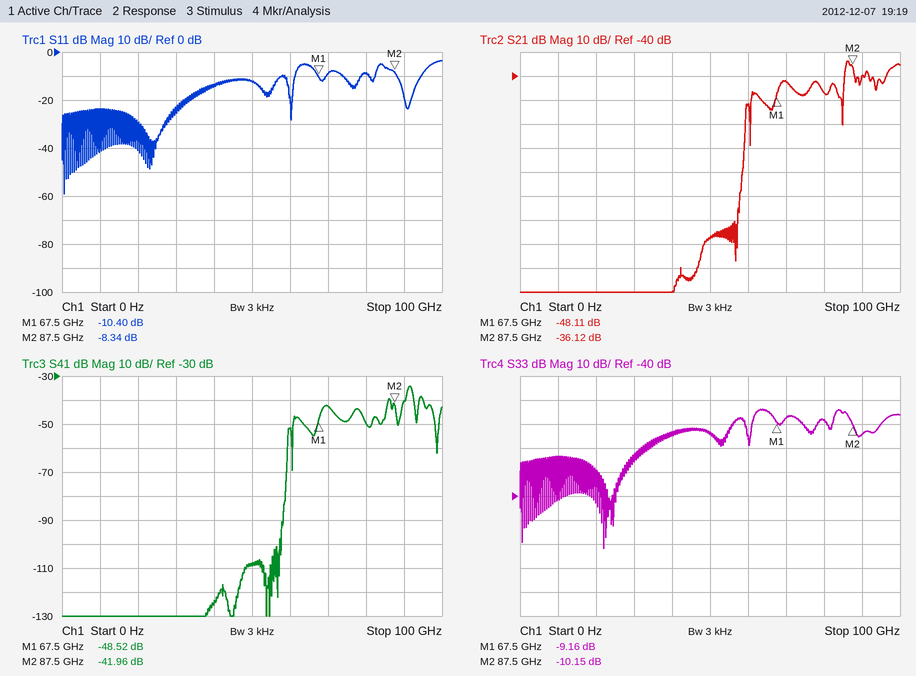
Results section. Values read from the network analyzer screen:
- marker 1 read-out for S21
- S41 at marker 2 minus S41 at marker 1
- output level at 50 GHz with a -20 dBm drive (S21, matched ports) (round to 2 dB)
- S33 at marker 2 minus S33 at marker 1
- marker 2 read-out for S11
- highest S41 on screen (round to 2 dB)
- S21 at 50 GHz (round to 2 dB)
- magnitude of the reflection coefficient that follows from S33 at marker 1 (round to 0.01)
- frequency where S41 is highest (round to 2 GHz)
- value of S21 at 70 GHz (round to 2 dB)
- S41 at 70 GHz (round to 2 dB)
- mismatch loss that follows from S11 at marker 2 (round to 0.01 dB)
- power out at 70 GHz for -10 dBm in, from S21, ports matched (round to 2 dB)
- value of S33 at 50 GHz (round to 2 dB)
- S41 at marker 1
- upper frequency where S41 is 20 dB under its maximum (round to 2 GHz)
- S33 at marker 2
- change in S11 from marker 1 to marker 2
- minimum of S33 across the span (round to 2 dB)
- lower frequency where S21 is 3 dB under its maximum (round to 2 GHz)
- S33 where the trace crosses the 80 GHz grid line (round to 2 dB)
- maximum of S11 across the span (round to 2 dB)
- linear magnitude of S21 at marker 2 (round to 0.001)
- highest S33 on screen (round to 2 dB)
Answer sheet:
-48.11 dB
6.56 dB
-128 dBm
-0.99 dB
-8.34 dB
-34 dB
-108 dB
0.35
92 GHz
-42 dB
-42 dB
0.69 dB
-52 dBm
-14 dB
-48.52 dB
98 GHz
-10.15 dB
2.06 dB
-62 dB
86 GHz
-8 dB
-4 dB
0.016
-4 dB
